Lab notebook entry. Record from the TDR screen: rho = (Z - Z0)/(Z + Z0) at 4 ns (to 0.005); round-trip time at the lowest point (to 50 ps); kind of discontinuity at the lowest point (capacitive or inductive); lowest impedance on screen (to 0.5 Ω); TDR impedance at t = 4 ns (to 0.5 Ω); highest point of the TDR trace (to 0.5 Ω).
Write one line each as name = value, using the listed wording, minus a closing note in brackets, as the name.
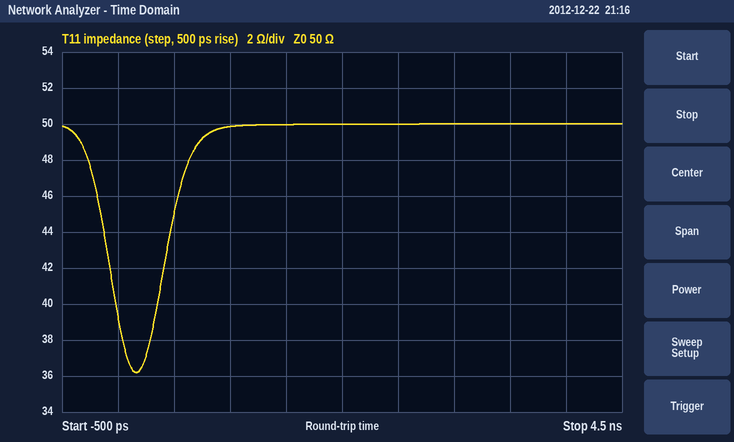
rho = (Z - Z0)/(Z + Z0) at 4 ns = 0.000
round-trip time at the lowest point = 150 ps
kind of discontinuity at the lowest point = capacitive
lowest impedance on screen = 36.0 Ω
TDR impedance at t = 4 ns = 50.0 Ω
highest point of the TDR trace = 50.0 Ω
